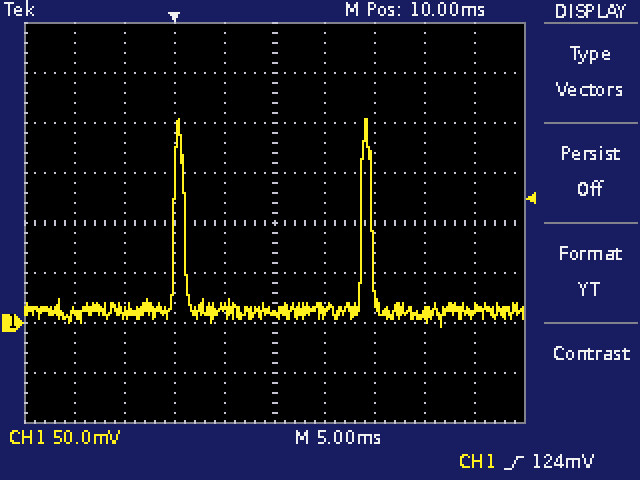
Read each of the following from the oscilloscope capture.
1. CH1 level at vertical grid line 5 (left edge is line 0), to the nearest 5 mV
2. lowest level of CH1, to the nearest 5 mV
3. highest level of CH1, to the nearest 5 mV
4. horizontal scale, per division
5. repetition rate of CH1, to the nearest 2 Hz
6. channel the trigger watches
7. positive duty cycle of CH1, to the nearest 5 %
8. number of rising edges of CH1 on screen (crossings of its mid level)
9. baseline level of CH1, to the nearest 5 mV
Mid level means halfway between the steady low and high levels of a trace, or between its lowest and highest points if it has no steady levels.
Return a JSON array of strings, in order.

["10 mV", "-5 mV", "205 mV", "5 ms", "54 Hz", "CH1", "5 %", "2", "10 mV"]
